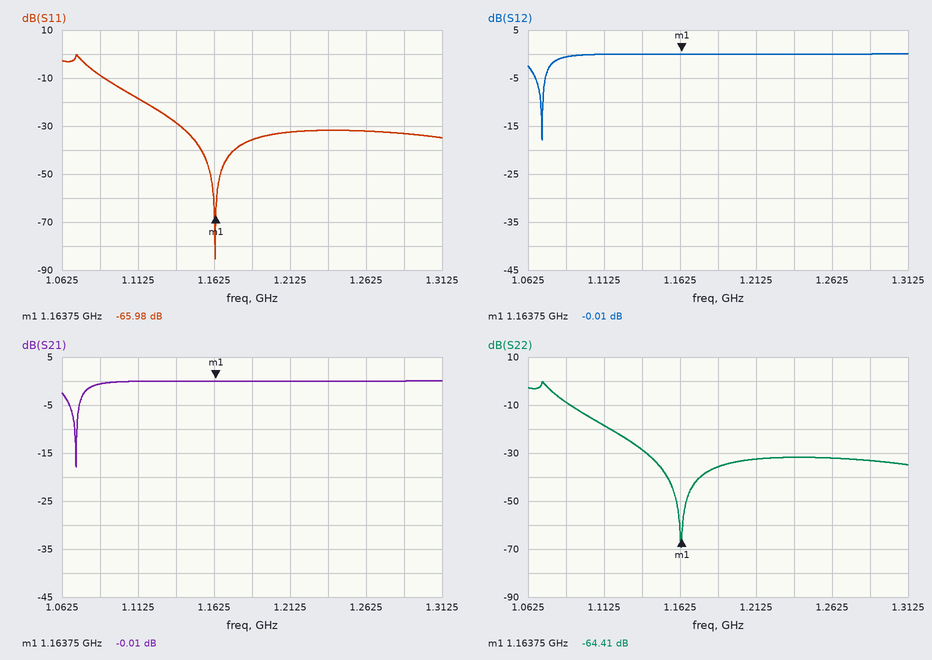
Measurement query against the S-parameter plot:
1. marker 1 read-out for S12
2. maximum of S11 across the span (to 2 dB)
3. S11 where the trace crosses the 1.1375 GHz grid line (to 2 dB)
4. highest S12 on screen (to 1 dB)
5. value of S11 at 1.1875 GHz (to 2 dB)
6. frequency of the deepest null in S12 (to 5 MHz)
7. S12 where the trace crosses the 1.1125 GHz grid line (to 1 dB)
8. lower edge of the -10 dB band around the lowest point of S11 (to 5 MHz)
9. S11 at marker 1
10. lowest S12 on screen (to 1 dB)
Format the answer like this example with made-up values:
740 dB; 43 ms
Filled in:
-0.01 dB; 0 dB; -28 dB; 0 dB; -36 dB; 1.070 GHz; 0 dB; 1.090 GHz; -65.98 dB; -18 dB
